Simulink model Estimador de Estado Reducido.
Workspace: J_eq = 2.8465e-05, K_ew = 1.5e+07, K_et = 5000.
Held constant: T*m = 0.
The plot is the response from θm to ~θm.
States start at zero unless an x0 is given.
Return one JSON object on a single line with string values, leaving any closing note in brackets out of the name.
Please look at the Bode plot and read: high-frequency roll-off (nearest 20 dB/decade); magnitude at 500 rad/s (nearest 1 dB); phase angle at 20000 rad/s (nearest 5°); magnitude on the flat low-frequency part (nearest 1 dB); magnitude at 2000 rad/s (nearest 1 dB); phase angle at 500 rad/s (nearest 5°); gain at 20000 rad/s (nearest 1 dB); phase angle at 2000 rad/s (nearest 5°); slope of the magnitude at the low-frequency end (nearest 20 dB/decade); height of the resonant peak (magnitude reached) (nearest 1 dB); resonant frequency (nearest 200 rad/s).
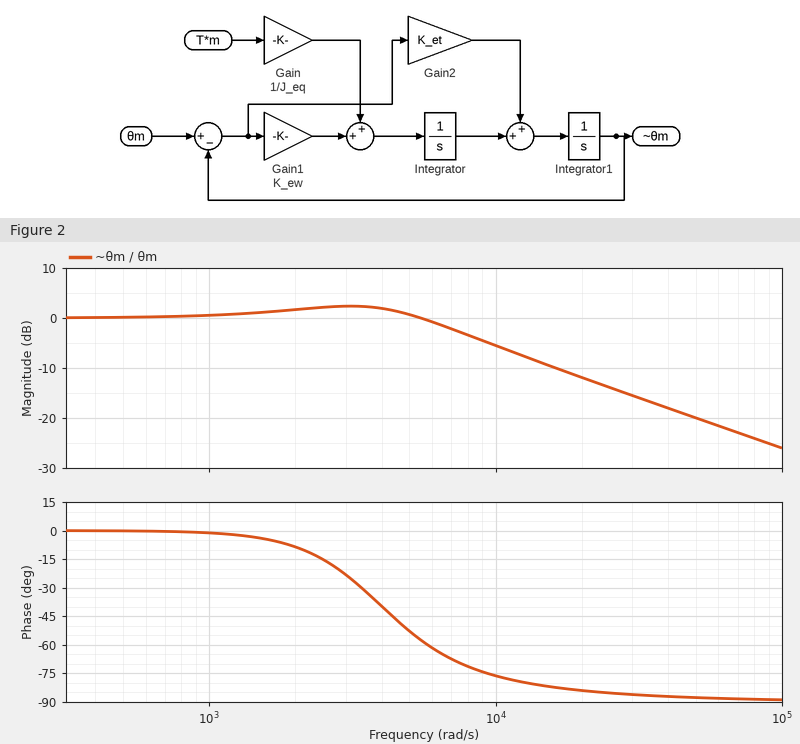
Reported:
{"high-frequency roll-off": "-20 dB/decade", "magnitude at 500 rad/s": "0 dB", "phase angle at 20000 rad/s": "-85°", "magnitude on the flat low-frequency part": "0 dB", "magnitude at 2000 rad/s": "2 dB", "phase angle at 500 rad/s": "0°", "gain at 20000 rad/s": "-12 dB", "phase angle at 2000 rad/s": "-10°", "slope of the magnitude at the low-frequency end": "0 dB/decade", "height of the resonant peak (magnitude reached)": "2 dB", "resonant frequency": "3000 rad/s"}
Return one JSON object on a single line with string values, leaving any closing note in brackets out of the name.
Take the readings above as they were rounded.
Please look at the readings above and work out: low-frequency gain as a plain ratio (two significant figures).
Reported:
{"low-frequency gain as a plain ratio": "1.0"}
